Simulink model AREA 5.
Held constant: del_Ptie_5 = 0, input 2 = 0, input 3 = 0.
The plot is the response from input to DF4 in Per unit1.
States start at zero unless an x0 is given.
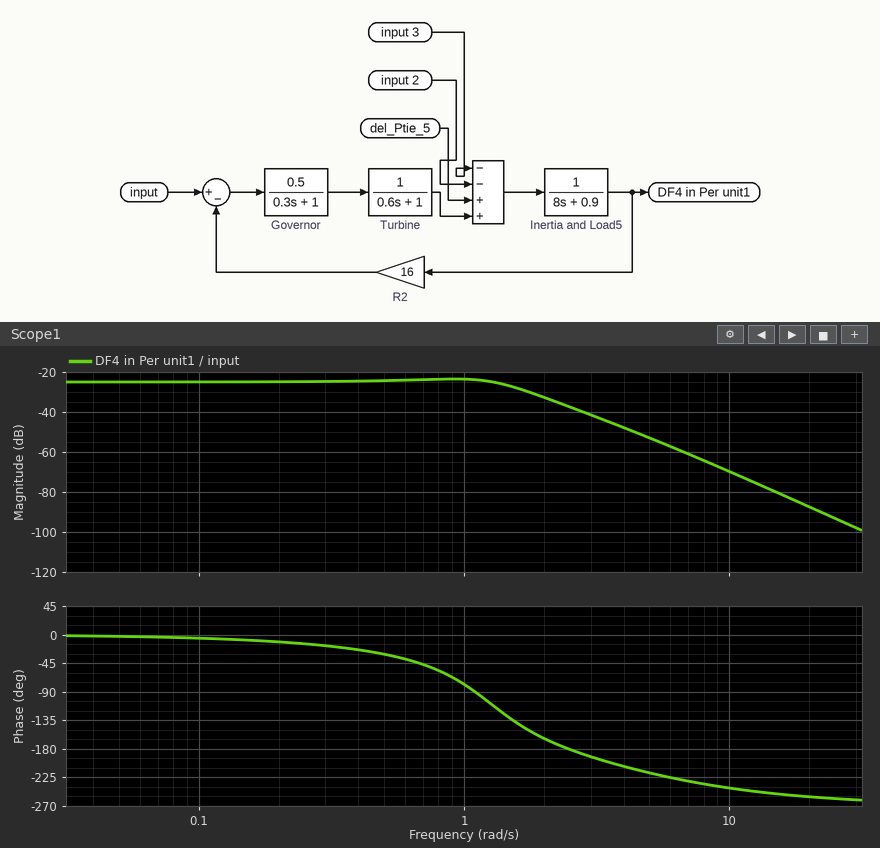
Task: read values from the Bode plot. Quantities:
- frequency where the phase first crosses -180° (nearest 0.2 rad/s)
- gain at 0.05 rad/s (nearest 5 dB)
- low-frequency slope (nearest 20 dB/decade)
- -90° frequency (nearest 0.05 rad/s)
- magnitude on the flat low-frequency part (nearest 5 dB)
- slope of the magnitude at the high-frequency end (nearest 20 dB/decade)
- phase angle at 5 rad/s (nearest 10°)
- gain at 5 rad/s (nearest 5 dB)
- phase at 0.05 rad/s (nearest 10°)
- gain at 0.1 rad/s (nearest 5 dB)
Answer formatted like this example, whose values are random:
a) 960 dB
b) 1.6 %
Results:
a) 2.4 rad/s
b) -25 dB
c) 0 dB/decade
d) 1.10 rad/s
e) -25 dB
f) -60 dB/decade
g) -220°
h) -55 dB
i) 0°
j) -25 dB
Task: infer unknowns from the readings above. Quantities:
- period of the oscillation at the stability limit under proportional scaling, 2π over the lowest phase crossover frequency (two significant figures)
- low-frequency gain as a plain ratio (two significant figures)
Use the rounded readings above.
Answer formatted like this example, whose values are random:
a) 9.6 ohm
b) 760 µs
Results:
a) 2.6 s
b) 0.056
